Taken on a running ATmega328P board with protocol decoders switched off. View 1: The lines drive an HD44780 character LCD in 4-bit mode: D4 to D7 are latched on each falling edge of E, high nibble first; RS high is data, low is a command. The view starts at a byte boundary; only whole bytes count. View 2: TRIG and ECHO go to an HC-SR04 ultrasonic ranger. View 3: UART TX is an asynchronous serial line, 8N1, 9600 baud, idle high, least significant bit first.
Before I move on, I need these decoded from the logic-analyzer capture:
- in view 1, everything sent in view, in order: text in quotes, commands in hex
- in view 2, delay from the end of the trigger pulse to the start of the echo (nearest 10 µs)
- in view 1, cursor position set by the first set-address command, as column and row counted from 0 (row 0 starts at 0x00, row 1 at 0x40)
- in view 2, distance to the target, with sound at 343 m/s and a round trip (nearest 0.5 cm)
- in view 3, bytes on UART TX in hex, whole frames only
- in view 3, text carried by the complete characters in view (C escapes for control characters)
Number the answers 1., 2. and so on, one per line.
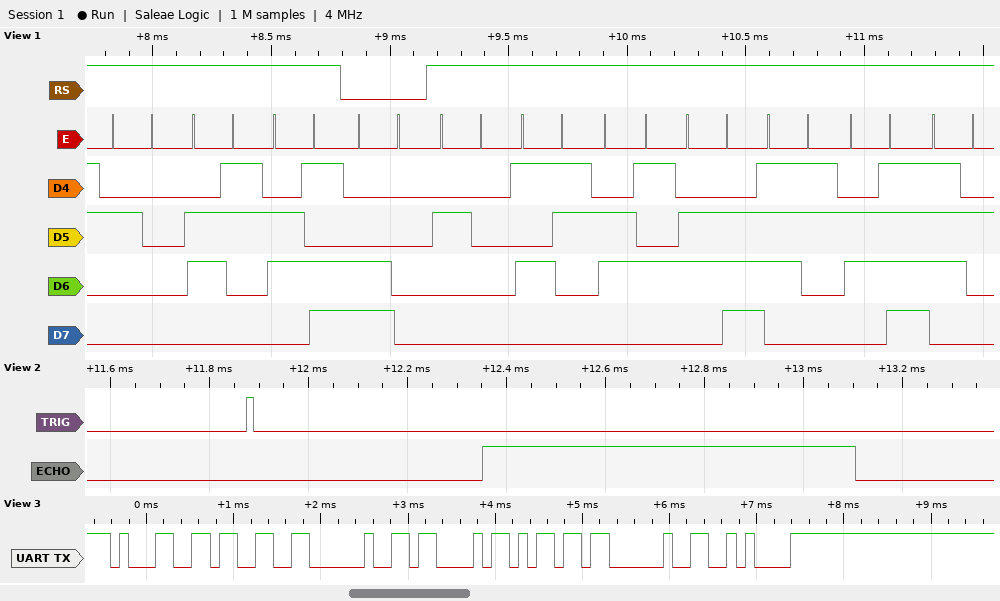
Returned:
1. " cm" 0xC0 " Sensor"
2. 460 µs
3. column 0, row 1
4. 13 cm
5. 31 33 20 43 6D 20 0A
6. "13 Cm \n"
